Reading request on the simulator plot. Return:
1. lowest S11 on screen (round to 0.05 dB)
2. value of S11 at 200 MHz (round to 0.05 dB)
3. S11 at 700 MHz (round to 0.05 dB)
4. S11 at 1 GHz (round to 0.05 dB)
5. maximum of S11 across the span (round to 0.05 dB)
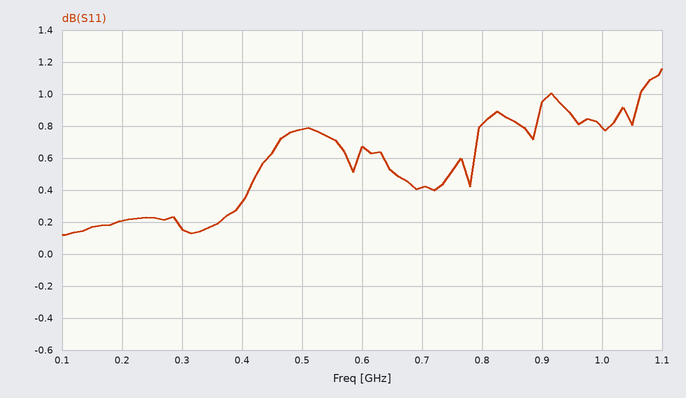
0.10 dB
0.20 dB
0.40 dB
0.80 dB
1.15 dB
